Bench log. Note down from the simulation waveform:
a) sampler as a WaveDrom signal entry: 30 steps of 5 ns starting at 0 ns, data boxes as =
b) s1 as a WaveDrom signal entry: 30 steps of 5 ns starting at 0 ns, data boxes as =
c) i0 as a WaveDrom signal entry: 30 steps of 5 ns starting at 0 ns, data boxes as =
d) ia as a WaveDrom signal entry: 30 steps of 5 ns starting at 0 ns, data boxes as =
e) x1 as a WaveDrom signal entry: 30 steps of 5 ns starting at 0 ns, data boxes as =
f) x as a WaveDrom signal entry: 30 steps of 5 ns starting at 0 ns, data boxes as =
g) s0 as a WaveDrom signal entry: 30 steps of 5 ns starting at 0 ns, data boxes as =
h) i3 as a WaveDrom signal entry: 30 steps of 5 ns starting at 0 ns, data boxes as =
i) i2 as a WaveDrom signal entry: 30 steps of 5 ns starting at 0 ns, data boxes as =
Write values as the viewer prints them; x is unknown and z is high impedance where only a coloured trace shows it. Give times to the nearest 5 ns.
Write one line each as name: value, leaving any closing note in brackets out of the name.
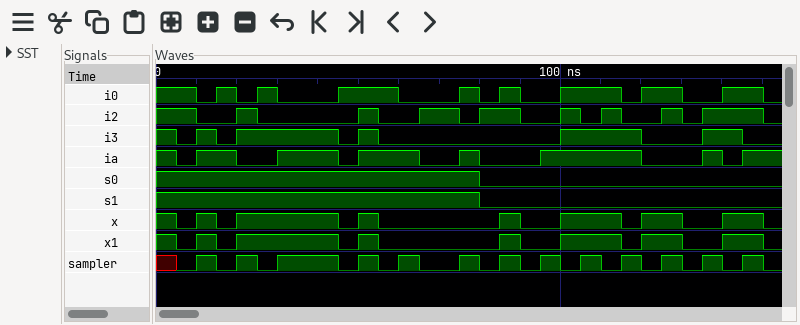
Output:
sampler as a WaveDrom signal entry: 30 steps of 5 ns starting at 0 ns, data boxes as =: {name: 'sampler', wave: 'x010101..01010.101010101010101'}
s1 as a WaveDrom signal entry: 30 steps of 5 ns starting at 0 ns, data boxes as =: {name: 's1', wave: '1...............0.............'}
i0 as a WaveDrom signal entry: 30 steps of 5 ns starting at 0 ns, data boxes as =: {name: 'i0', wave: '1.01010..1..0..1010.1..01.0.1.'}
ia as a WaveDrom signal entry: 30 steps of 5 ns starting at 0 ns, data boxes as =: {name: 'ia', wave: '101.0.1..01..0.10..1....0..101'}
x1 as a WaveDrom signal entry: 30 steps of 5 ns starting at 0 ns, data boxes as =: {name: 'x1', wave: '10101....010.....10.1..01.0.1.'}
x as a WaveDrom signal entry: 30 steps of 5 ns starting at 0 ns, data boxes as =: {name: 'x', wave: '10101....010.....10.1..01.0.1.'}
s0 as a WaveDrom signal entry: 30 steps of 5 ns starting at 0 ns, data boxes as =: {name: 's0', wave: '1...............0.............'}
i3 as a WaveDrom signal entry: 30 steps of 5 ns starting at 0 ns, data boxes as =: {name: 'i3', wave: '10101....010........1...0..1.0'}
i2 as a WaveDrom signal entry: 30 steps of 5 ns starting at 0 ns, data boxes as =: {name: 'i2', wave: '1.0.10....10.1.01.0.1010.101..'}
